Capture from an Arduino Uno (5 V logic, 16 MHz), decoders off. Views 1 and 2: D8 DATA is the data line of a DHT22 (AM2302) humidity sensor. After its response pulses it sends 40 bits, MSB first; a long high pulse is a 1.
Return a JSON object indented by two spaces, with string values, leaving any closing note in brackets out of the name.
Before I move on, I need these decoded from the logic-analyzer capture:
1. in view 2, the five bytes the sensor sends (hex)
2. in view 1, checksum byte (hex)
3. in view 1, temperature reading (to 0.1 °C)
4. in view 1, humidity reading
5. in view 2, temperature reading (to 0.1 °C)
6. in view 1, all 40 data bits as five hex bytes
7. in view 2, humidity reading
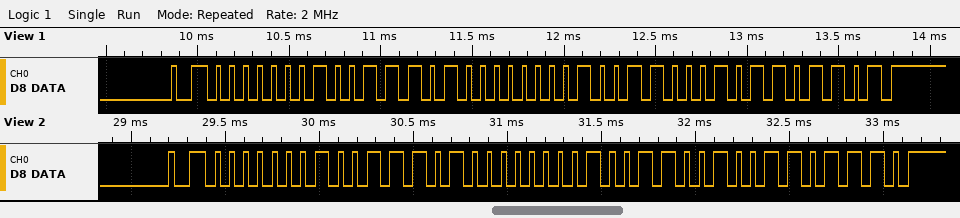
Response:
{
  "in view 2, the five bytes the sensor sends": "01 3A 01 32 6E",
  "in view 1, checksum byte": "0x6D",
  "in view 1, temperature reading": "30.5 °C",
  "in view 1, humidity reading": "31.4 %",
  "in view 2, temperature reading": "30.6 °C",
  "in view 1, all 40 data bits as five hex bytes": "01 3A 01 31 6D",
  "in view 2, humidity reading": "31.4 %"
}
